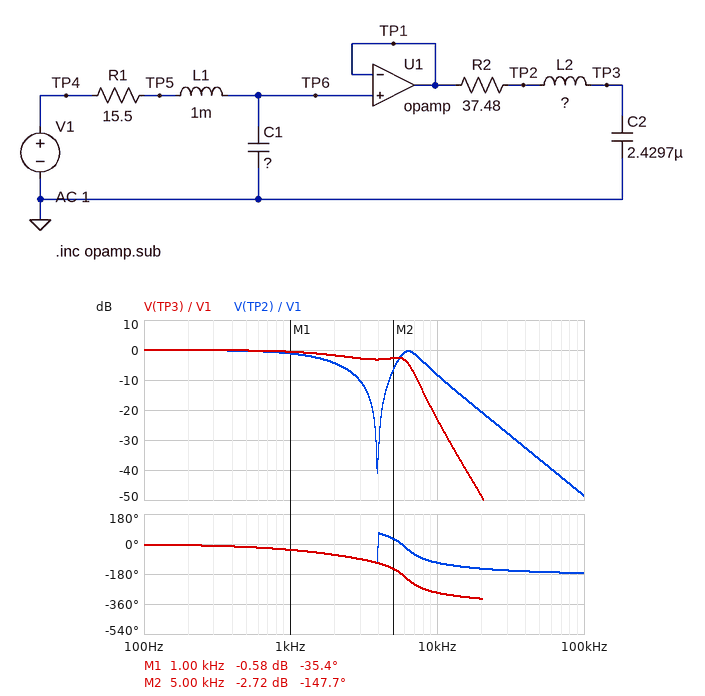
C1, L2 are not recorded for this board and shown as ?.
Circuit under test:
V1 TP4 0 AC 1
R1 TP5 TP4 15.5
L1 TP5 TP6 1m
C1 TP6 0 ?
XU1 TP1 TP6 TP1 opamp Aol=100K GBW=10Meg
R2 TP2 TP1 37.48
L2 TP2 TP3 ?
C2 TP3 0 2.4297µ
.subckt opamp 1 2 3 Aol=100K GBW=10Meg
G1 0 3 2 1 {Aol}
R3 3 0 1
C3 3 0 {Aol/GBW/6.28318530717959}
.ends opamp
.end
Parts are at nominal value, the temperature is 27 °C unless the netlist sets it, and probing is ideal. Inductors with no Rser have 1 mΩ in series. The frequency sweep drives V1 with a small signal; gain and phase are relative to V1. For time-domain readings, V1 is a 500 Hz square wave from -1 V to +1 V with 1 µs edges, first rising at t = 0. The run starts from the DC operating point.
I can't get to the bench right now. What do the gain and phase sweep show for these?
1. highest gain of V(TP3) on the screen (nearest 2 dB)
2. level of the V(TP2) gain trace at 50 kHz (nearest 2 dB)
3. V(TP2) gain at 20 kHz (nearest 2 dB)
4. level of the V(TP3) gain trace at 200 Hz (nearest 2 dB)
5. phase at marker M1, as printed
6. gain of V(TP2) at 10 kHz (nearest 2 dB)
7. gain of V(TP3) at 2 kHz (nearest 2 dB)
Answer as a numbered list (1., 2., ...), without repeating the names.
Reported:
1. 0 dB
2. -36 dB
3. -20 dB
4. 0 dB
5. -35.4 deg
6. -8 dB
7. -2 dB
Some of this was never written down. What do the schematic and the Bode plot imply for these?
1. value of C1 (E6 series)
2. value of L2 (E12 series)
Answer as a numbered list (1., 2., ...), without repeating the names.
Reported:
1. 680 nF
2. 680 µH
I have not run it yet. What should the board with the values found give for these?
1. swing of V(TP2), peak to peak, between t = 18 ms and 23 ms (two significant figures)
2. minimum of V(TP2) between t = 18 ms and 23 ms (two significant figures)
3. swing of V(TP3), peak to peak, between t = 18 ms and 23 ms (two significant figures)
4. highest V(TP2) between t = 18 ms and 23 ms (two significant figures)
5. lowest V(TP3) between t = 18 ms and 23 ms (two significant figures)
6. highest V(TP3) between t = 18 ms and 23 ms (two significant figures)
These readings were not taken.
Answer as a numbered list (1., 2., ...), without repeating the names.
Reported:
1. 2.1 V
2. -1.0 V
3. 2.1 V
4. 1.0 V
5. -1.0 V
6. 1.0 V
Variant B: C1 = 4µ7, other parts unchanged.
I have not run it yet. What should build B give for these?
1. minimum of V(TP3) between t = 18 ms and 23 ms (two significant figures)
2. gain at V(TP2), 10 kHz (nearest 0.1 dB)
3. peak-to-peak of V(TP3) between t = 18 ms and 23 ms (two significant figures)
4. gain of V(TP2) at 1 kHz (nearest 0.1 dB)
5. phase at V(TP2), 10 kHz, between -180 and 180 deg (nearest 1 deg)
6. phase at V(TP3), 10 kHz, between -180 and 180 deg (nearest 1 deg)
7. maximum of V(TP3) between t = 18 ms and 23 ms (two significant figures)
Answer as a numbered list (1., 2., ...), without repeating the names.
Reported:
1. -1.1 V
2. -28.3 dB
3. 2.3 V
4. -0.8 dB
5. -119 deg
6. 61 deg
7. 1.1 V
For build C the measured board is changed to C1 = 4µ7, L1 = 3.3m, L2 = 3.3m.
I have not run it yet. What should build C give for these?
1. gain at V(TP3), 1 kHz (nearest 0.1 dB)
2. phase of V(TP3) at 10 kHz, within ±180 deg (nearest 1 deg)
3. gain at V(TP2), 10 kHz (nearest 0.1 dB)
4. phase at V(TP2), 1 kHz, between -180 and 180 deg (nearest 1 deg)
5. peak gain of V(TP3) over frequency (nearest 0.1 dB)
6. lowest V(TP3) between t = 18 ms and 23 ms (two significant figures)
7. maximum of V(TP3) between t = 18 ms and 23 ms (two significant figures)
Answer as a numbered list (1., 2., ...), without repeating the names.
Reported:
1. 5.4 dB
2. 15 deg
3. -35.8 dB
4. -90 deg
5. 6.2 dB
6. -1.9 V
7. 1.9 V
